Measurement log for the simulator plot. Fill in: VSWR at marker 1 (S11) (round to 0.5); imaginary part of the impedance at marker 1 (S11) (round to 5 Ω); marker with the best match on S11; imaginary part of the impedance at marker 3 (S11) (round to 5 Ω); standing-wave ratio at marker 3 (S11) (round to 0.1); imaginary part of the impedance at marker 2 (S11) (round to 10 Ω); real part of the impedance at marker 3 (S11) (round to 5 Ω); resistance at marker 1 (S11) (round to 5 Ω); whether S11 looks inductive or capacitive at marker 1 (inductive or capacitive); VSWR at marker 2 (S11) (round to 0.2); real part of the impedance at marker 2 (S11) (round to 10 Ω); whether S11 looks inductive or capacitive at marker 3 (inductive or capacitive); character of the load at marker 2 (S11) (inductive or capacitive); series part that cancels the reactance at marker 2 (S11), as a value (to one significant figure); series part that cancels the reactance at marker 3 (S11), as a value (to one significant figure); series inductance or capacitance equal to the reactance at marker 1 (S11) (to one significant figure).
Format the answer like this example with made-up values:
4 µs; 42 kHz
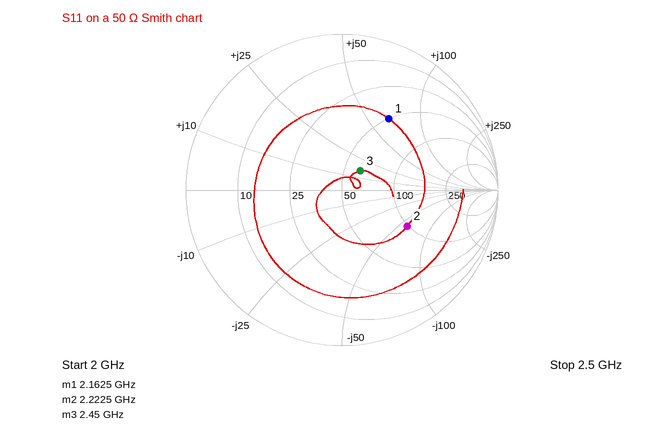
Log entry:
3.5; +65 Ω; marker 3; +15 Ω; 1.4; -60 Ω; 60 Ω; 50 Ω; inductive; 2.8; 100 Ω; inductive; capacitive; 4 nH; 4 pF; 5 nH
